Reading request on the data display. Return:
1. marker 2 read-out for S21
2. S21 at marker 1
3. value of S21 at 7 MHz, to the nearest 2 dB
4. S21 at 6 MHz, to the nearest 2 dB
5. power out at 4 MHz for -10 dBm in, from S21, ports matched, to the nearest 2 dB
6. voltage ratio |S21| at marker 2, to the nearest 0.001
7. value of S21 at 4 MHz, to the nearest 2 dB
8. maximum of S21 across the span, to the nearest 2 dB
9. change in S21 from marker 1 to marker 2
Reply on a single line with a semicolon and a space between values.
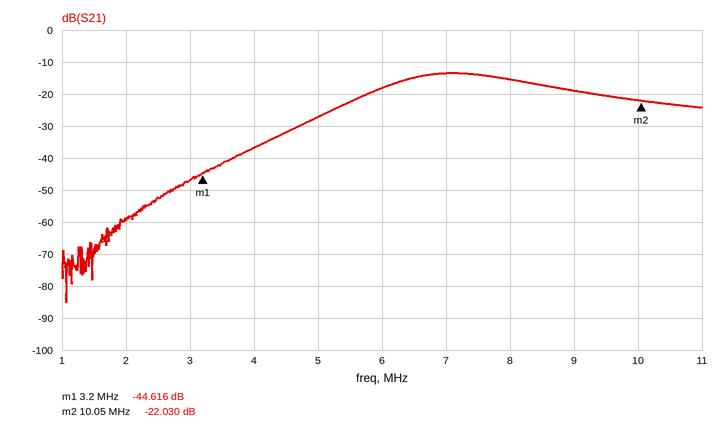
-22.030 dB; -44.616 dB; -14 dB; -18 dB; -46 dBm; 0.079; -36 dB; -14 dB; 22.586 dB
